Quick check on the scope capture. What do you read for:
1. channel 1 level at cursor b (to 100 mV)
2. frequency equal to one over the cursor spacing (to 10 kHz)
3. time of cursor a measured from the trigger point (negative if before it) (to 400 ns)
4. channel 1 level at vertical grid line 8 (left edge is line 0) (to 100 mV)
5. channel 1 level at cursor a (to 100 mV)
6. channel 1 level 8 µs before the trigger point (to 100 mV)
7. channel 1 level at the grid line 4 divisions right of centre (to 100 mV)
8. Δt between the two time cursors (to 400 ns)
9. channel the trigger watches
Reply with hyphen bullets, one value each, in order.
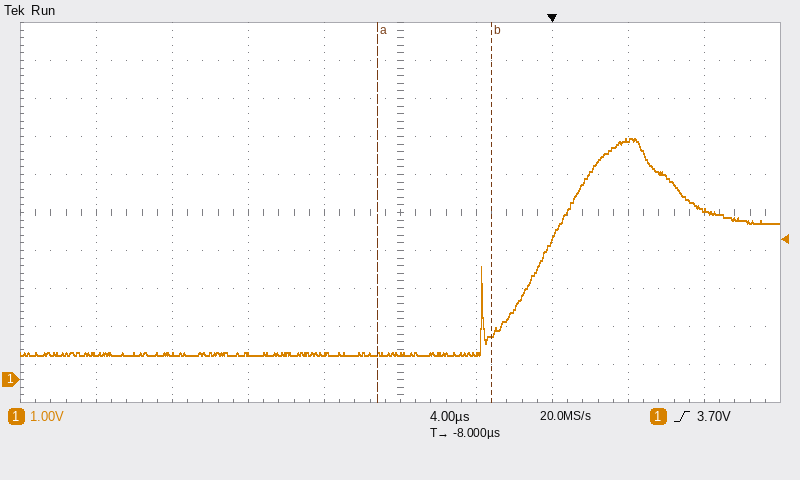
- 1.2 V
- 170 kHz
- -9.2 µs
- 6.3 V
- 700 mV
- 700 mV
- 4.5 V
- 6.0 µs
- channel 1
